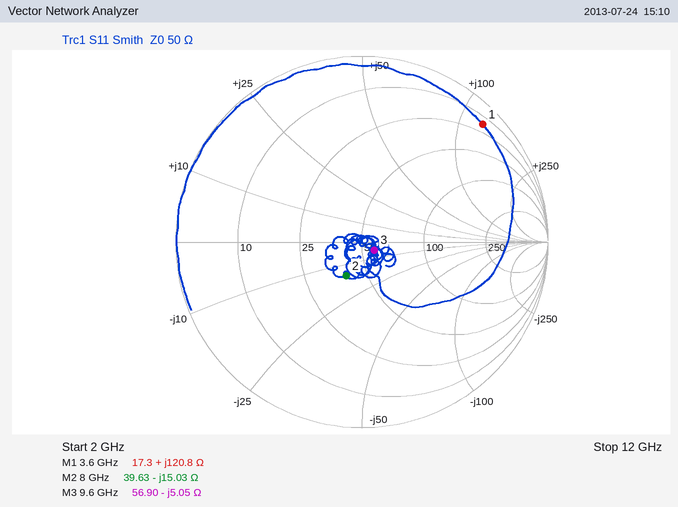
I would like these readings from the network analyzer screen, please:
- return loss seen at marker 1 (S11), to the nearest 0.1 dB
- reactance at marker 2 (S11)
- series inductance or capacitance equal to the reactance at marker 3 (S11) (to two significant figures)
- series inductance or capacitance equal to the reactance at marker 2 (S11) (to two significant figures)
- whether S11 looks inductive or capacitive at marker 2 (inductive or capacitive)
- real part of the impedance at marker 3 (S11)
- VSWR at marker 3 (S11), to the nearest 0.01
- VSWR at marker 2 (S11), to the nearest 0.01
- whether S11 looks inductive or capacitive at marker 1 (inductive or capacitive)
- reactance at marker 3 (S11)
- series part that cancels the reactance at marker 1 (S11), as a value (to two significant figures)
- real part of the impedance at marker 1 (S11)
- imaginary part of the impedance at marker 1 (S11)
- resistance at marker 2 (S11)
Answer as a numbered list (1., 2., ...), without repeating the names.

1. 0.9 dB
2. -15.03 Ω
3. 3.3 pF
4. 1.3 pF
5. capacitive
6. 56.90 Ω
7. 1.17
8. 1.50
9. inductive
10. -5.05 Ω
11. 370 fF
12. 17.3 Ω
13. +120.8 Ω
14. 39.63 Ω
